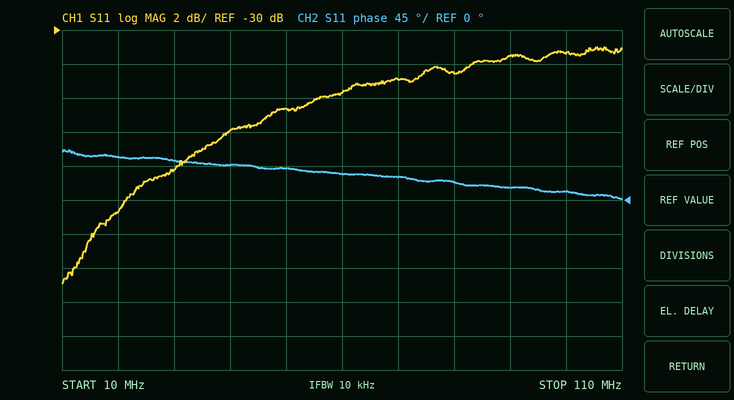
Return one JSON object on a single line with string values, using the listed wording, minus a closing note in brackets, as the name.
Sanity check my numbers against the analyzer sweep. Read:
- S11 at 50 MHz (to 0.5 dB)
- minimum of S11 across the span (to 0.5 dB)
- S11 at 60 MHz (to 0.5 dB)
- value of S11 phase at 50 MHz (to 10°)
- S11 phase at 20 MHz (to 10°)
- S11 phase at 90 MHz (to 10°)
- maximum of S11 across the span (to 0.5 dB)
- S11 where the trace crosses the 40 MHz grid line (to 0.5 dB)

{"S11 at 50 MHz": "-34.5 dB", "minimum of S11 across the span": "-45.0 dB", "S11 at 60 MHz": "-33.5 dB", "value of S11 phase at 50 MHz": "40°", "S11 phase at 20 MHz": "60°", "S11 phase at 90 MHz": "20°", "maximum of S11 across the span": "-31.0 dB", "S11 where the trace crosses the 40 MHz grid line": "-36.0 dB"}
